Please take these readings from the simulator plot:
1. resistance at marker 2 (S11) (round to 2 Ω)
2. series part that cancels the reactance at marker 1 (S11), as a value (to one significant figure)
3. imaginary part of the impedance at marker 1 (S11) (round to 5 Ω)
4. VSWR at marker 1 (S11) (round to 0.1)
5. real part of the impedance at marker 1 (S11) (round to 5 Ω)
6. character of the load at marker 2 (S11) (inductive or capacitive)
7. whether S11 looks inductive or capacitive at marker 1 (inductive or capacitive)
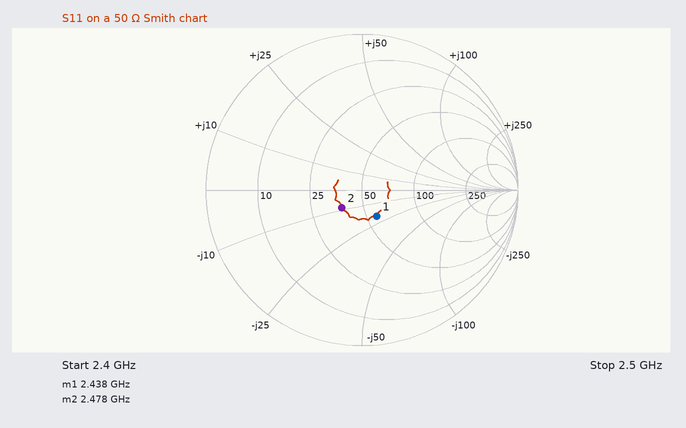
38 Ω
1 nH
-20 Ω
1.5
55 Ω
capacitive
capacitive
